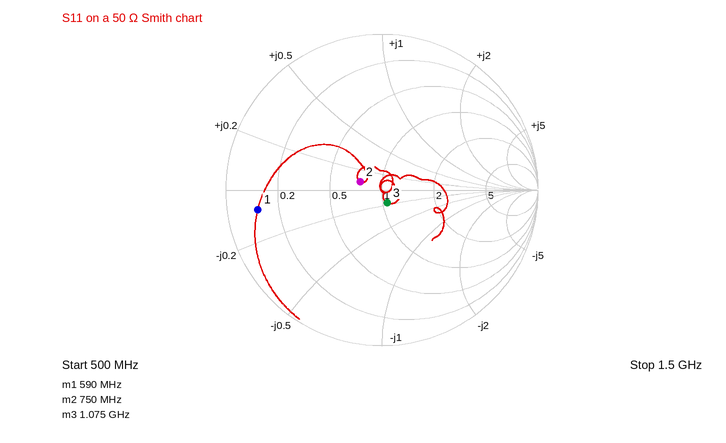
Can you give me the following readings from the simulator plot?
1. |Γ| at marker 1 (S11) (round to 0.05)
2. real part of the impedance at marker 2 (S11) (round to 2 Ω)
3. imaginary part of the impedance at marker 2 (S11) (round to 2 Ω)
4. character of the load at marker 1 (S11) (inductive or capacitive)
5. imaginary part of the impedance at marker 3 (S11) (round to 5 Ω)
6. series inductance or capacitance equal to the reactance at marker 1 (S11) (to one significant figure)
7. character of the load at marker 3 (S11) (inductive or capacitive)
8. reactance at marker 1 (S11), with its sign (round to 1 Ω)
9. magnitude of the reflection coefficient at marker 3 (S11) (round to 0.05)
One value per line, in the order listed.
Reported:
0.80
38 Ω
+4 Ω
capacitive
-10 Ω
70 pF
capacitive
-4 Ω
0.10
